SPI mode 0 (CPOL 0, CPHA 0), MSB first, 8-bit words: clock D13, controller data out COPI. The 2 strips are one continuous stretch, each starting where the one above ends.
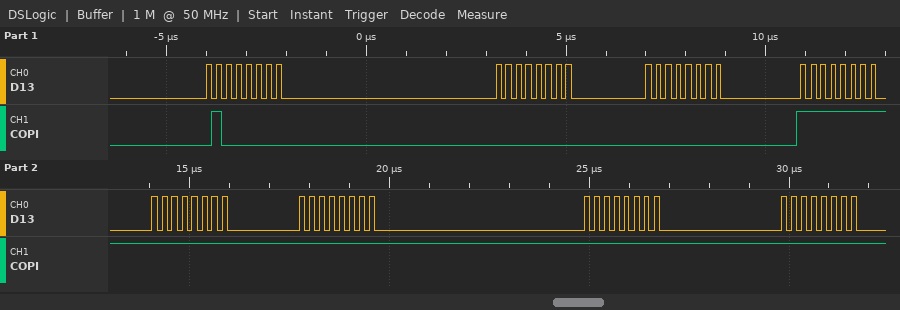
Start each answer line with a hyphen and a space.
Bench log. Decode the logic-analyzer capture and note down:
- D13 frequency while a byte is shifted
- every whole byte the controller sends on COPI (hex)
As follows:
- 4 MHz
- 40 00 00 FF FF FF FF FF
